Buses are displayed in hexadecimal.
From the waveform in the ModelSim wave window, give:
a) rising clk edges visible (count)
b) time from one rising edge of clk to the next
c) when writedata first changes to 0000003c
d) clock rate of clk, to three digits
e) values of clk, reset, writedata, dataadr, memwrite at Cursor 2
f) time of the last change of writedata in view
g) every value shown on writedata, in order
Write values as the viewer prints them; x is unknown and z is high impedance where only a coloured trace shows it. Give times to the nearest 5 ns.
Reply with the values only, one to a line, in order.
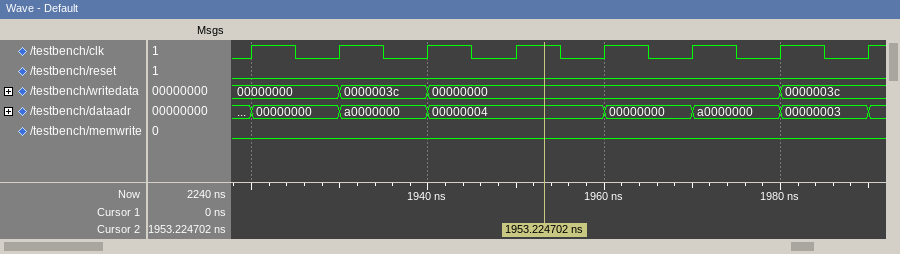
8
10 ns
1930 ns
100 MHz
clk=1, reset=0, writedata=00000000, dataadr=00000004, memwrite=0
1980 ns
00000000, 0000003c, 00000000, 0000003c
